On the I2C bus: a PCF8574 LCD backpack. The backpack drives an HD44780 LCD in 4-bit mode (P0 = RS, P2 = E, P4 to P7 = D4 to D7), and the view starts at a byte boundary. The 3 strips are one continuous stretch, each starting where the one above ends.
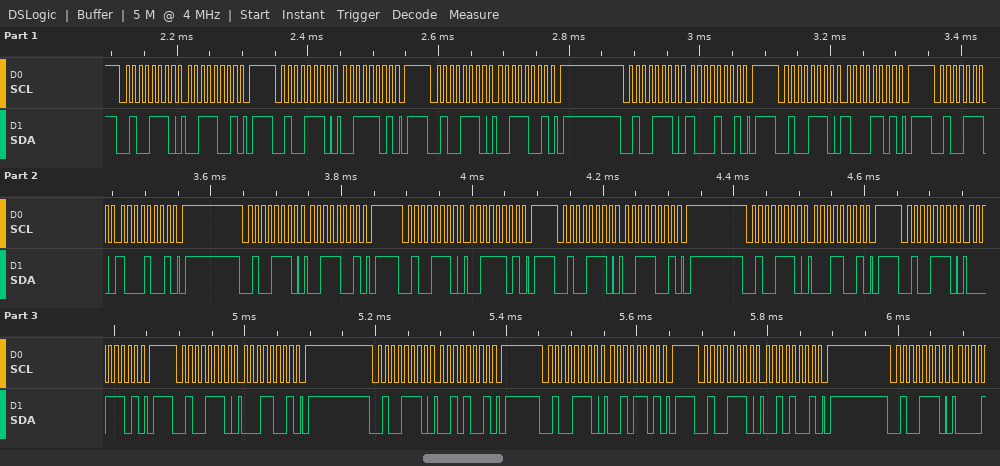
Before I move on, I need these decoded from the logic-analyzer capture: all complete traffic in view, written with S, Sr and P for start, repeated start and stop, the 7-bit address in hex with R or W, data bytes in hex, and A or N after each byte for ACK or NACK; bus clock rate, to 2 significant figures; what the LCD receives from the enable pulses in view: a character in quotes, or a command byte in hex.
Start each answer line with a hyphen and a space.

- S 27W A 39 A P S 27W A 3D A P S 27W A 39 A P S 27W A 89 A P S 27W A 8D A P S 27W A 89 A P S 27W A 39 A P S 27W A 3D A P S 27W A 39 A P S 27W A 19 A P S 27W A 1D A P S 27W A 19 A P S 27W A 29 A P S 27W A 2D A P S 27W A 29 A P S 27W A
- 100 kHz
- '8' '1'
